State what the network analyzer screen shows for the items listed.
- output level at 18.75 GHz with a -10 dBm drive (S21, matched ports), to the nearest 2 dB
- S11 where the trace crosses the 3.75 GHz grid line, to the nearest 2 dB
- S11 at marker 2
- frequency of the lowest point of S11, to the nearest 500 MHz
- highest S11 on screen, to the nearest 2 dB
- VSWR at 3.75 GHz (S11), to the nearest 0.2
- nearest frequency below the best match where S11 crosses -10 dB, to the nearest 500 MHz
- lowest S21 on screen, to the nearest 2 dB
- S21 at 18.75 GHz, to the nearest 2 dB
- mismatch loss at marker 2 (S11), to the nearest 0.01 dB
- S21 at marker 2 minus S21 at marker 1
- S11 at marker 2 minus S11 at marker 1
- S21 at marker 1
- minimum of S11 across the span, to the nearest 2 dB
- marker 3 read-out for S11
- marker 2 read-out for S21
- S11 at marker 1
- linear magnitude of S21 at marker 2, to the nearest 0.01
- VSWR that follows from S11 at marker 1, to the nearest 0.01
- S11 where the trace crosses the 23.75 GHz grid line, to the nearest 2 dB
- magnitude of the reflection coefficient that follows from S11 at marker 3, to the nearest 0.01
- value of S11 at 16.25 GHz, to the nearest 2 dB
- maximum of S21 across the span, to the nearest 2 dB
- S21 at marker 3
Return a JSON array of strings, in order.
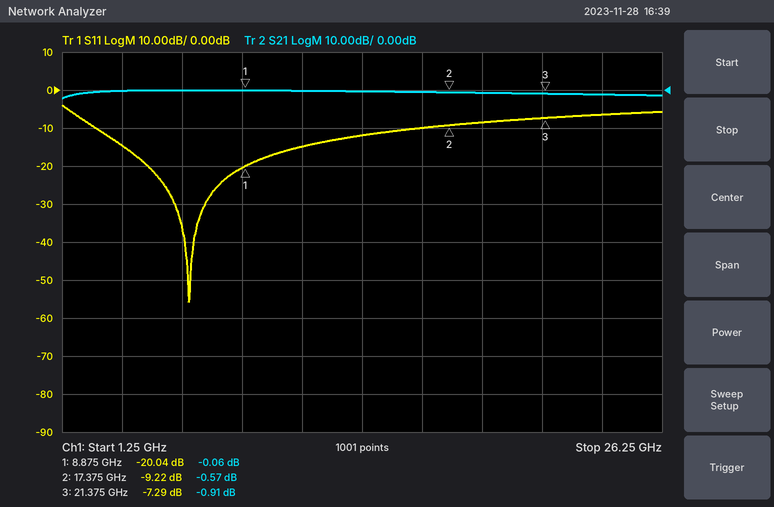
["-10 dBm", "-14 dB", "-9.22 dB", "6.5 GHz", "-4 dB", "1.4", "2.5 GHz", "-2 dB", "0 dB", "0.55 dB", "-0.51 dB", "10.82 dB", "-0.06 dB", "-56 dB", "-7.29 dB", "-0.57 dB", "-20.04 dB", "0.94", "1.22", "-6 dB", "0.43", "-10 dB", "0 dB", "-0.91 dB"]
